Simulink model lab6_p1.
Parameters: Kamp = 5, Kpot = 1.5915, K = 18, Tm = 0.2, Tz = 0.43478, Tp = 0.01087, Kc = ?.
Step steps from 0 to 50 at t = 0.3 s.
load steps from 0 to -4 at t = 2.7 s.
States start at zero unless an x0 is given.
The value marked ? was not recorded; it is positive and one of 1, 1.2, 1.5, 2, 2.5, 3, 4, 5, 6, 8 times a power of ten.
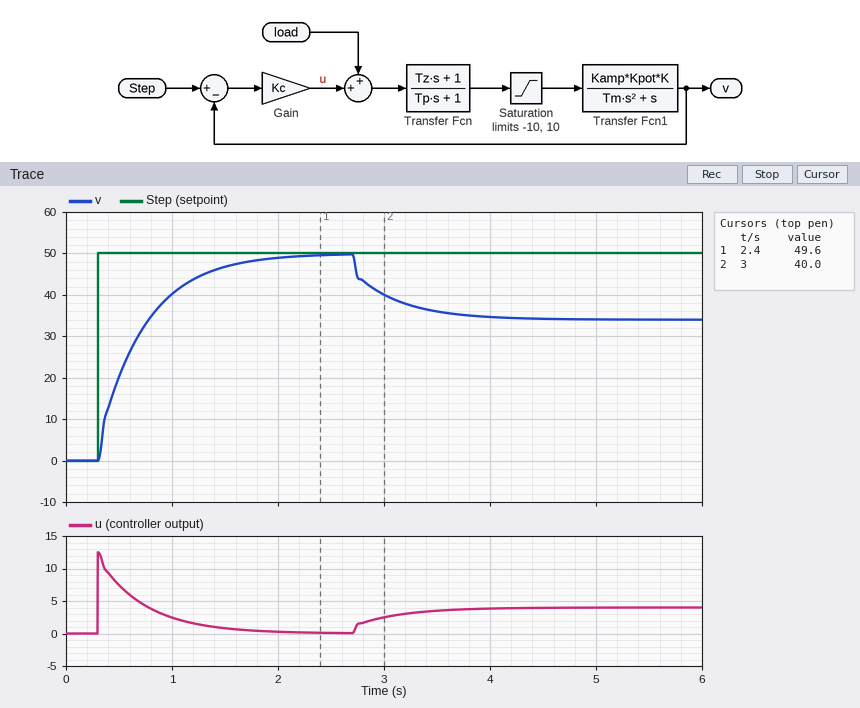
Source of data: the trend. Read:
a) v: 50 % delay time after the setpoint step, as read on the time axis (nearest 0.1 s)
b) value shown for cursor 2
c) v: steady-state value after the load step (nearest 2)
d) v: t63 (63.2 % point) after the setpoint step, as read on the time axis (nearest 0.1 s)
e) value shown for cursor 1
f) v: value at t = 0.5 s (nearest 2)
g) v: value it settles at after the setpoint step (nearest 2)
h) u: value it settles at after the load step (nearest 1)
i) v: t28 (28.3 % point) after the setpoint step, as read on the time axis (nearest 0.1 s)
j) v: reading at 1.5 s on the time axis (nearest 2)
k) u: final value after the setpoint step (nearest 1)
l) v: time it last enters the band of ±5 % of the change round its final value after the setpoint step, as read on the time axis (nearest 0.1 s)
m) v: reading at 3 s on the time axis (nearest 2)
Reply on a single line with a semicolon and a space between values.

0.6 s; 40.0; 34; 0.7 s; 49.6; 20; 50; 4; 0.4 s; 46; 0; 1.6 s; 40
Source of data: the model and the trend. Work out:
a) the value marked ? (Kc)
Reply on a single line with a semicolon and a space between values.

0.25
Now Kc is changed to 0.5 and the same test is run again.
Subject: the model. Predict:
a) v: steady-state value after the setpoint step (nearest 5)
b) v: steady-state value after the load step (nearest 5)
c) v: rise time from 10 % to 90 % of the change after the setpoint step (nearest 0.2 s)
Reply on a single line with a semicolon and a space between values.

50; 40; 1.0 s
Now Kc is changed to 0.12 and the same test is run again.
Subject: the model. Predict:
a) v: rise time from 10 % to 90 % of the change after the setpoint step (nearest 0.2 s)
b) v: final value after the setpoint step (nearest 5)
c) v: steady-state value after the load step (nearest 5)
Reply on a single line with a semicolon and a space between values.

1.0 s; 50; 15
